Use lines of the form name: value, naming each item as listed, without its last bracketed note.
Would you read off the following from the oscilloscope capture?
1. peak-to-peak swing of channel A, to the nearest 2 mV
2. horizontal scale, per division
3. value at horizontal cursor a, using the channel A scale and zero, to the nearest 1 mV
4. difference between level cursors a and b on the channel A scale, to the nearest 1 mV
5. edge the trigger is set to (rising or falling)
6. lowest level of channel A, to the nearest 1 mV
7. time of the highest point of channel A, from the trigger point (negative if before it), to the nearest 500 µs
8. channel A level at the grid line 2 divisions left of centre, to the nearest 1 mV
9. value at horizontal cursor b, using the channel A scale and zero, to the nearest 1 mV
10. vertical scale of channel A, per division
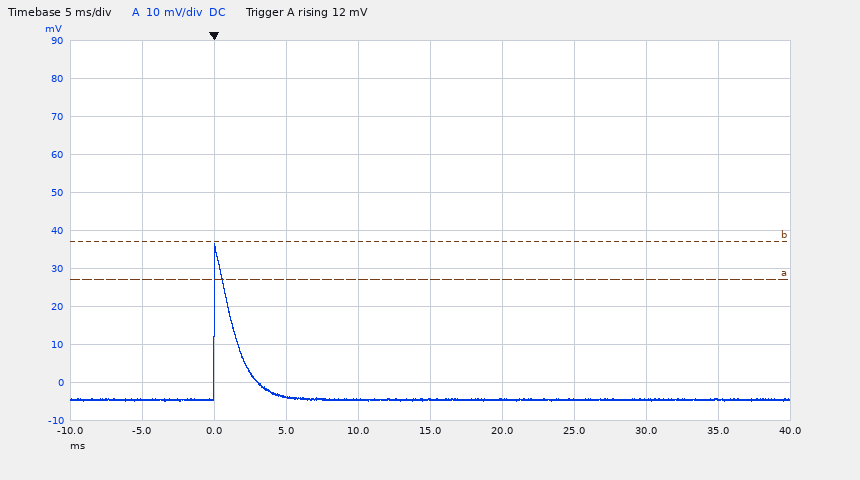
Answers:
peak-to-peak swing of channel A, to the nearest 2 mV: 42 mV
horizontal scale, per division: 5 ms
value at horizontal cursor a, using the channel A scale and zero, to the nearest 1 mV: 27 mV
difference between level cursors a and b on the channel A scale, to the nearest 1 mV: 10 mV
edge the trigger is set to: rising
lowest level of channel A, to the nearest 1 mV: -5 mV
time of the highest point of channel A, from the trigger point (negative if before it), to the nearest 500 µs: 0.0 ms
channel A level at the grid line 2 divisions left of centre, to the nearest 1 mV: -4 mV
value at horizontal cursor b, using the channel A scale and zero, to the nearest 1 mV: 37 mV
vertical scale of channel A, per division: 10 mV
